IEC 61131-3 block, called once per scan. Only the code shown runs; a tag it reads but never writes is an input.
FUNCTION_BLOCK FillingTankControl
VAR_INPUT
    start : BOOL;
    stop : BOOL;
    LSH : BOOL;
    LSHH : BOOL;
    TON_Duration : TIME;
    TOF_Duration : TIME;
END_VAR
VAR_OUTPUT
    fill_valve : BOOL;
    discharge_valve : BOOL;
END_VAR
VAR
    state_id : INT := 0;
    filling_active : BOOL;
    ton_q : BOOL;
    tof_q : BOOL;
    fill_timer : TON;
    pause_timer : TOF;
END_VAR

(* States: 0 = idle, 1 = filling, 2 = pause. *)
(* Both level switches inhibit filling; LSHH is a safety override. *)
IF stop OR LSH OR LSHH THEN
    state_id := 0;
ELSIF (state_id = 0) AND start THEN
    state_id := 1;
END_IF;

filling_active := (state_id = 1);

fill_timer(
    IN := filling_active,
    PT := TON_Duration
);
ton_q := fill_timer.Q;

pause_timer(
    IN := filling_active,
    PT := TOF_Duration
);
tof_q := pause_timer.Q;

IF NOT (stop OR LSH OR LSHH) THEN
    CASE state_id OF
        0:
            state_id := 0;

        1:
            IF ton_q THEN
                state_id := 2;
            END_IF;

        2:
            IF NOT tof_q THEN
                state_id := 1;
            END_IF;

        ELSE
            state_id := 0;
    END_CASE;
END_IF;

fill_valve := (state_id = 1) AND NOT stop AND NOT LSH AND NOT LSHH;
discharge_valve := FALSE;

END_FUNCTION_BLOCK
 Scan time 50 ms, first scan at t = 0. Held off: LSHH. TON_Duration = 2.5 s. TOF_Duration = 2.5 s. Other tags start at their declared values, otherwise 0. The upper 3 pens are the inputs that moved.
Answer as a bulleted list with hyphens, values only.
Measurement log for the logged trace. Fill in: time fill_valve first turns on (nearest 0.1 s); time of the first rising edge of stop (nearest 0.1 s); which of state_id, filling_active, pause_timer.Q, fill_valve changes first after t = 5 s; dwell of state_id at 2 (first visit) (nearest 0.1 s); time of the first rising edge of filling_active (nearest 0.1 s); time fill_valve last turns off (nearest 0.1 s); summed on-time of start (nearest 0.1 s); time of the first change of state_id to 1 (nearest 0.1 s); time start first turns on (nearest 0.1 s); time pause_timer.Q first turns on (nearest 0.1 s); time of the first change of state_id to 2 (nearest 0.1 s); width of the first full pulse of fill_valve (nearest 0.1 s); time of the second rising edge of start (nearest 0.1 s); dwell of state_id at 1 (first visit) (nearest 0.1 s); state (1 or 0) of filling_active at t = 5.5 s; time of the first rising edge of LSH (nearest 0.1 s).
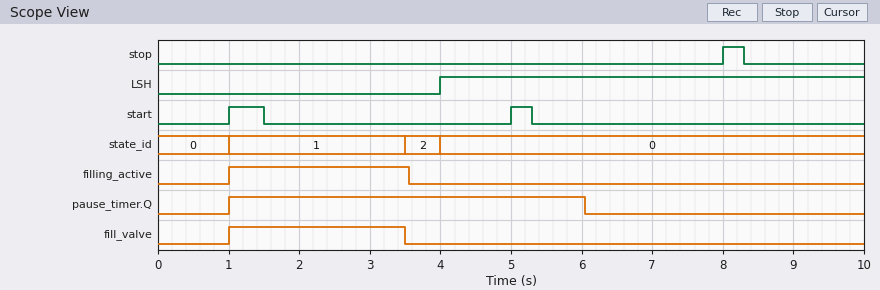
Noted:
- 1.0 s
- 8.0 s
- pause_timer.Q
- 0.5 s
- 1.0 s
- 3.5 s
- 0.8 s
- 1.0 s
- 1.0 s
- 1.0 s
- 3.5 s
- 2.5 s
- 5.0 s
- 2.5 s
- 0
- 4.0 s
